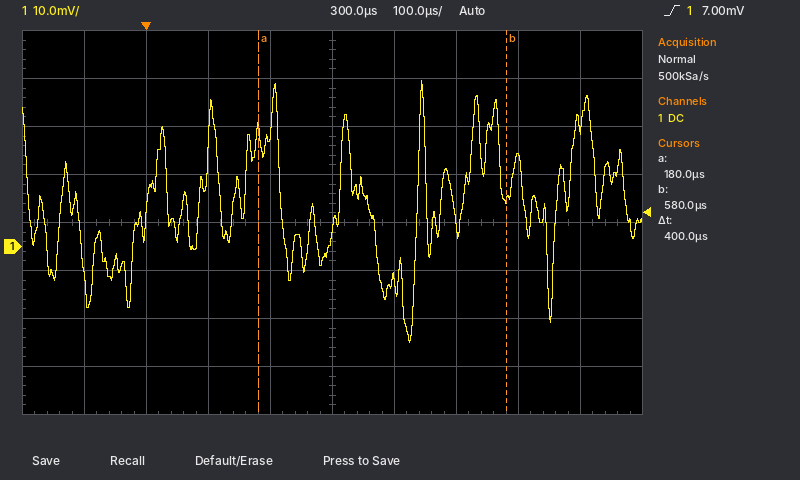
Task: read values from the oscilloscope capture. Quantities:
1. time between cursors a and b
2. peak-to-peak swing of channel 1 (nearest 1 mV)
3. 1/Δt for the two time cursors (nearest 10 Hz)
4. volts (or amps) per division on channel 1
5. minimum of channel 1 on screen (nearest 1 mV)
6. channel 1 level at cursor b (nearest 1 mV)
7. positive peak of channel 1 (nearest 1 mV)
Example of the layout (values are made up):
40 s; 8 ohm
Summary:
400 µs; 55 mV; 2.50 kHz; 10 mV; -20 mV; 10 mV; 35 mV
